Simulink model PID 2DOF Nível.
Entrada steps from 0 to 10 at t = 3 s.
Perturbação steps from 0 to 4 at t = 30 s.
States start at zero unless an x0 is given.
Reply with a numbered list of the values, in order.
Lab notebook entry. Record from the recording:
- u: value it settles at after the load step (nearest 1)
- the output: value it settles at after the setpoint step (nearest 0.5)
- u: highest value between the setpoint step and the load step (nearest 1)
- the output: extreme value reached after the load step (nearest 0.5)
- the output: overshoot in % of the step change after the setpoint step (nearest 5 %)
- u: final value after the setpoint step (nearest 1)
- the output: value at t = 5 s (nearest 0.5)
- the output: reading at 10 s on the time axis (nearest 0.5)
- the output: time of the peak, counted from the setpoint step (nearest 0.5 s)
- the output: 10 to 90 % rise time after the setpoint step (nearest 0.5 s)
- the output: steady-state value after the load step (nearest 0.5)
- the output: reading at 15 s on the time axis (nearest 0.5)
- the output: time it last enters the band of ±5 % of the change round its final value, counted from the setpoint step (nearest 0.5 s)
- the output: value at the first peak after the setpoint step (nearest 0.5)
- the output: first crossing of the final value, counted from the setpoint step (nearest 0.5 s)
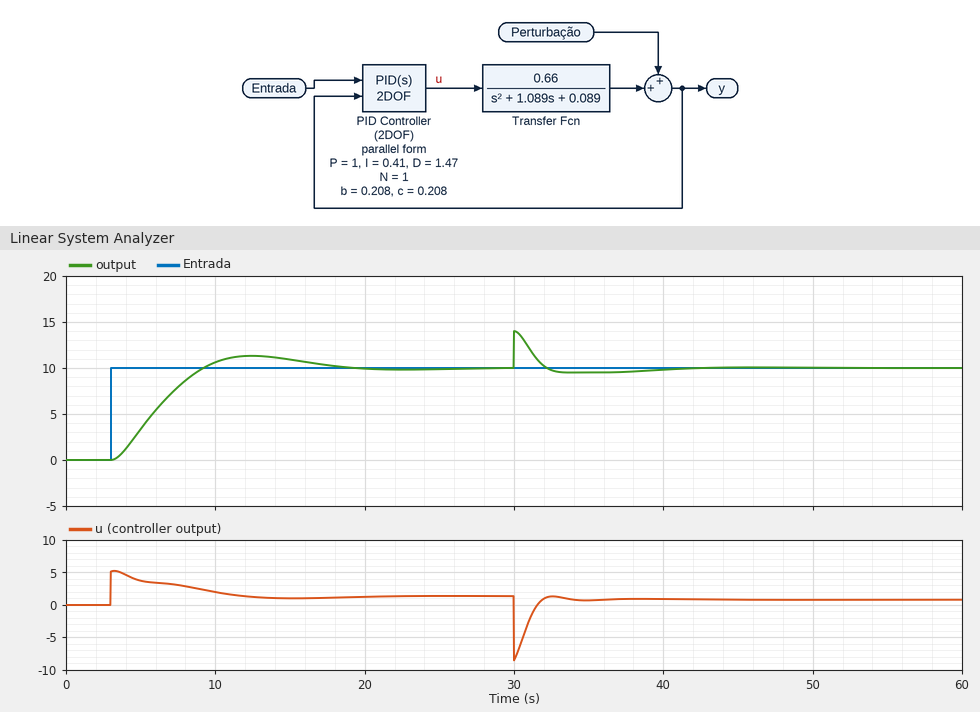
1. 1
2. 10.0
3. 5
4. 14.0
5. 15 %
6. 1
7. 3.5
8. 10.5
9. 9.5 s
10. 4.5 s
11. 10.0
12. 11.0
13. 13.5 s
14. 11.5
15. 6.0 s
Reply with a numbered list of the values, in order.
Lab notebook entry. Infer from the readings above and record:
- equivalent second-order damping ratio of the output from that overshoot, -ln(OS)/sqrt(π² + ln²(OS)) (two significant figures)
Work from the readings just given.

1. 0.52
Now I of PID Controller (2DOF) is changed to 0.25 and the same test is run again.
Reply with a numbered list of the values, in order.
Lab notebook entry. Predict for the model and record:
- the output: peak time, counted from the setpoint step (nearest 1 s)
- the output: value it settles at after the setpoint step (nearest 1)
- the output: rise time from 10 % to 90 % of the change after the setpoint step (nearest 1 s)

1. 14 s
2. 10
3. 7 s
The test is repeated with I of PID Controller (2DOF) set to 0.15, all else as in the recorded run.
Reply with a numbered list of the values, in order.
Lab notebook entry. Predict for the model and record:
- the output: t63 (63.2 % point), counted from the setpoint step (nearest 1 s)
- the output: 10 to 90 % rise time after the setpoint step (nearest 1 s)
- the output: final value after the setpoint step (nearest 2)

1. 7 s
2. 12 s
3. 10
